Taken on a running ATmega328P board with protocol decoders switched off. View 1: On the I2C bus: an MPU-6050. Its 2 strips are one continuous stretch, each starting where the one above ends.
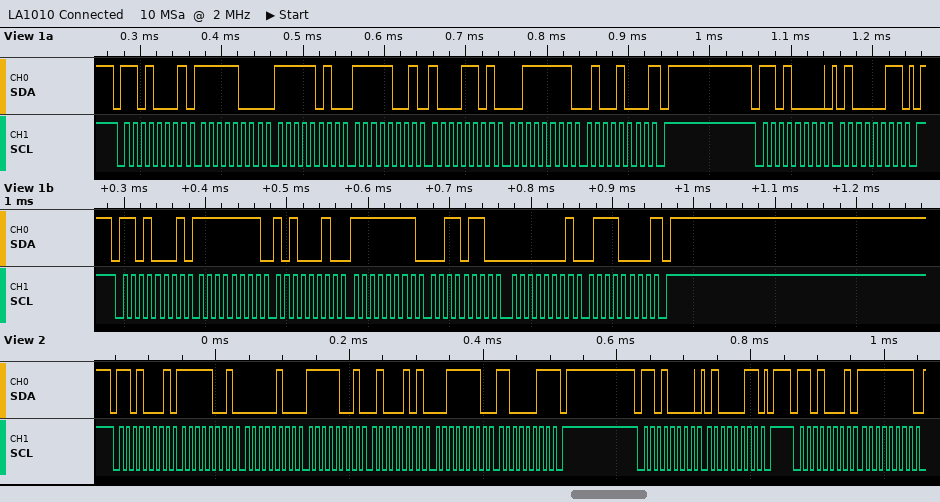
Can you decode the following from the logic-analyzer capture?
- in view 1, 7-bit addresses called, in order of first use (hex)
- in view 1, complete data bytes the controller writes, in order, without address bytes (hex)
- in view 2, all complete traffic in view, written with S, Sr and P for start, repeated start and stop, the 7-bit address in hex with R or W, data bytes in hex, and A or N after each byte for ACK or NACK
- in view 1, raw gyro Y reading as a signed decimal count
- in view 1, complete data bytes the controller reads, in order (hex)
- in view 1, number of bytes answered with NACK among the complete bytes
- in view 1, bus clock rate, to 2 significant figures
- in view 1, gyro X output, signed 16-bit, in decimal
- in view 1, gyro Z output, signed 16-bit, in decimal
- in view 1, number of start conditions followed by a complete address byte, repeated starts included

0x68
43
S 68R A F9 A 04 A F9 A 45 A 3E A C3 N P S 68W A 43 A P S 68R A FF A
-202
F8 FA F9 8D 3F 48 FF A2 FF 36 01 70
2
100 kHz
-94
368
3
